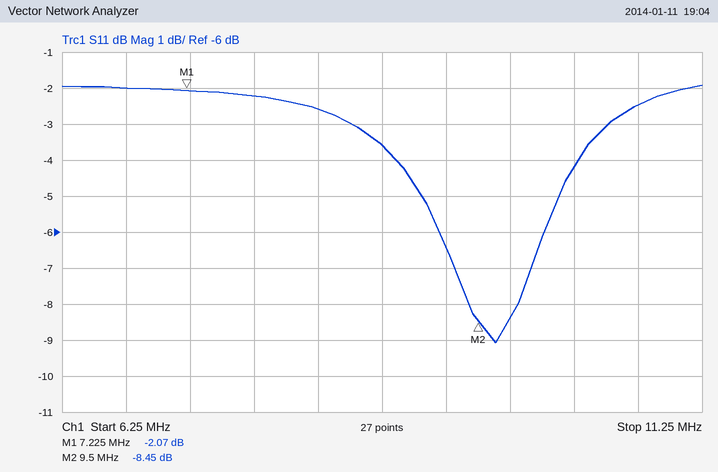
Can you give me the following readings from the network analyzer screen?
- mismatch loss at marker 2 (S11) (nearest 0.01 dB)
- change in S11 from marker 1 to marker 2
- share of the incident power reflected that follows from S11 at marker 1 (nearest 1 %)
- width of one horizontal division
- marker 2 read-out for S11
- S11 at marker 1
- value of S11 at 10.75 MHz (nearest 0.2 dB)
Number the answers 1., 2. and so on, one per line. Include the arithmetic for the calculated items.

1. −10 log10(1 − 10^(-8.45/10)) ≈ 0.67 dB
2. -8.45 − (-2.07) = -6.38 dB
3. 10^(-2.07/10) ≈ 62 %
4. 500 kHz
5. -8.45 dB
6. -2.07 dB
7. -2.4 dB
